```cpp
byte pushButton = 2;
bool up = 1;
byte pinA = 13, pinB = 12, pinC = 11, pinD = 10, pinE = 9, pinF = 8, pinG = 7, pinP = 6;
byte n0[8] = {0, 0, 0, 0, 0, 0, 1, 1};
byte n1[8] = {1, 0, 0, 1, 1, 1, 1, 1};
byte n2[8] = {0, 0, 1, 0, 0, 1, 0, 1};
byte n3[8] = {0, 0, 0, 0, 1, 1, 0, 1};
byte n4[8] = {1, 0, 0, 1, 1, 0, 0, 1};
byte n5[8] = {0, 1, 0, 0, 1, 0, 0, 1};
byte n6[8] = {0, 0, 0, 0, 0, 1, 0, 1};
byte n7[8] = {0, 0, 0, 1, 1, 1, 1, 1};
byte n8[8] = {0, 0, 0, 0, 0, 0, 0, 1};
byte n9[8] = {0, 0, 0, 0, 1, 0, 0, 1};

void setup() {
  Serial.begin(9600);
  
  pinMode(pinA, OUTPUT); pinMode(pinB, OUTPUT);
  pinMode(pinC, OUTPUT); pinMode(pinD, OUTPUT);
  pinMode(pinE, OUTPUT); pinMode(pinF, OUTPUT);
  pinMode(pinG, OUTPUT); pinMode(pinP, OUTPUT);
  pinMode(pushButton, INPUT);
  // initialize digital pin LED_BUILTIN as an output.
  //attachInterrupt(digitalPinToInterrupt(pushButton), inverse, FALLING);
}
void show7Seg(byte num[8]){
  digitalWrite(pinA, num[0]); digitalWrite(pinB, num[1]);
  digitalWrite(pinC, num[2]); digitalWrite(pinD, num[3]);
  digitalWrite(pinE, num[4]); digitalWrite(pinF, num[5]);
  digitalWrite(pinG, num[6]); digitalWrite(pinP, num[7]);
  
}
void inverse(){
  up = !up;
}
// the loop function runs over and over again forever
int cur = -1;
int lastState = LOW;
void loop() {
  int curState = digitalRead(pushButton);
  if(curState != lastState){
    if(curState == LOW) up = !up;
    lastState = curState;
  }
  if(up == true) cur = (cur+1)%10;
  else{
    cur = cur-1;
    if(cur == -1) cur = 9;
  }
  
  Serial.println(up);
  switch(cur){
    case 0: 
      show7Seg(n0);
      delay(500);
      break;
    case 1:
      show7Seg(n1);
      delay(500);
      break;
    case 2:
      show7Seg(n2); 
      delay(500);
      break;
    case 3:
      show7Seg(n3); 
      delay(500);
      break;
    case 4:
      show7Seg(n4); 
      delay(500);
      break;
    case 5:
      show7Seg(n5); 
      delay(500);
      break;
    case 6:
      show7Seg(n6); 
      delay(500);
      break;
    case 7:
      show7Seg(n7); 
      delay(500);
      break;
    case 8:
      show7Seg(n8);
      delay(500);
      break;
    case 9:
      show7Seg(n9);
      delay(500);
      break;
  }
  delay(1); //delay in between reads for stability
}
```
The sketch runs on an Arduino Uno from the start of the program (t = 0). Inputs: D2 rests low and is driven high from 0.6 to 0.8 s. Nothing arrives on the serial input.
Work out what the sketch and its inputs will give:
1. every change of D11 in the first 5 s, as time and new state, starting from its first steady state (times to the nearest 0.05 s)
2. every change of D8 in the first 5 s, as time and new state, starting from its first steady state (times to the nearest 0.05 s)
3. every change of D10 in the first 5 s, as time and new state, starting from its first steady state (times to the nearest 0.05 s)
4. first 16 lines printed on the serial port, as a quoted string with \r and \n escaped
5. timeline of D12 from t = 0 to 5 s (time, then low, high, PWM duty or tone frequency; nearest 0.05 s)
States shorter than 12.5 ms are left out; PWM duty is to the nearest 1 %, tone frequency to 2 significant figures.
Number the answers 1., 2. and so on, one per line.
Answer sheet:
1. 0 s low; 1 s high; 1.5 s low
2. 0 s low; 0.5 s high; 2 s low; 3 s high; 4 s low
3. 0 s low; 0.5 s high; 1 s low; 2 s high; 2.5 s low; 3.5 s high; 4 s low
4. "1\r\n1\r\n1\r\n1\r\n1\r\n1\r\n1\r\n1\r\n1\r\n1\r\n1\r\n1\r\n1\r\n1\r\n1\r\n1\r\n"
5. 0 s low; 2.5 s high; 3 s low
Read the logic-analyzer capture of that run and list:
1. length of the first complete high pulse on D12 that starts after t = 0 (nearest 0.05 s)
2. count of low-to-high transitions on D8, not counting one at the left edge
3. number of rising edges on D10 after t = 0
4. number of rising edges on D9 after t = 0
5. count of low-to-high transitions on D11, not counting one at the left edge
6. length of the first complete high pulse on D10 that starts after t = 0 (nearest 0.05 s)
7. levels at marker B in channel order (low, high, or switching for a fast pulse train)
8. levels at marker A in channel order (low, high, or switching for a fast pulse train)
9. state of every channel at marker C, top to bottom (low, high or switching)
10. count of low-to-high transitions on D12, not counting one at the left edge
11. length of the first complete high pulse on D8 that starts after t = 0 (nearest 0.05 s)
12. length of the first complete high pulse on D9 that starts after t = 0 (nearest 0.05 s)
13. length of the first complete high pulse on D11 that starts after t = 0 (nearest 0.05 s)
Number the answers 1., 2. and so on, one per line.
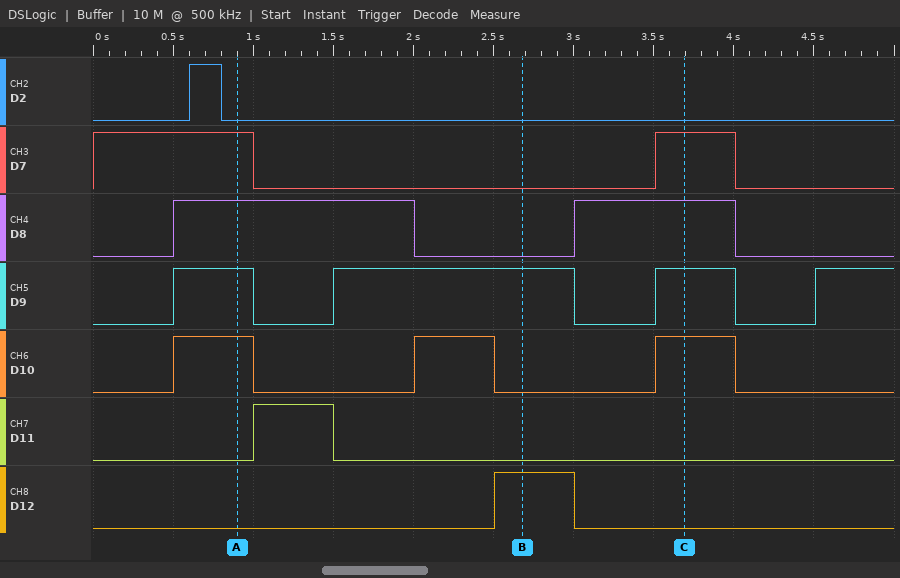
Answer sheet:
1. 0.50 s
2. 2
3. 3
4. 4
5. 1
6. 0.50 s
7. D2 low, D7 low, D8 low, D9 high, D10 low, D11 low, D12 high
8. D2 low, D7 high, D8 high, D9 high, D10 high, D11 low, D12 low
9. D2 low, D7 high, D8 high, D9 high, D10 high, D11 low, D12 low
10. 1
11. 1.50 s
12. 0.50 s
13. 0.50 s
